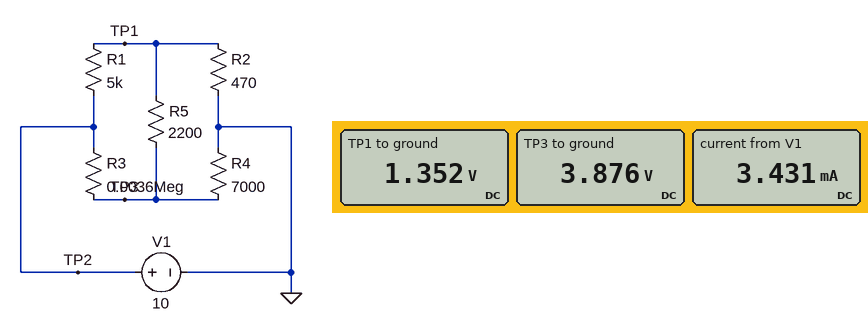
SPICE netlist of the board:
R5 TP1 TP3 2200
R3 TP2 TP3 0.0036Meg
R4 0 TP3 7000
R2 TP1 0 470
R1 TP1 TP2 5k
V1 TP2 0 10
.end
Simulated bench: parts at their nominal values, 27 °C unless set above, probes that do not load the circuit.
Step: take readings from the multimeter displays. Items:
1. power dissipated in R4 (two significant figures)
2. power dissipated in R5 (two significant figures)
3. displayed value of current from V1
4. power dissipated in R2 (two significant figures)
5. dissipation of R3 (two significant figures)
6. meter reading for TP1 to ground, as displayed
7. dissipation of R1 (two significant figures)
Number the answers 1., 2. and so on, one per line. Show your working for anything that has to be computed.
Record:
1. (3.876 V)^2 / 7 kΩ = 2.1 mW
2. (3.876 V - 1.352 V)^2 / 2.2 kΩ = 2.9 mW
3. 3.431 mA
4. (1.352 V)^2 / 470 Ω = 3.9 mW
5. (10 V - 3.876 V)^2 / 3.6 kΩ = 10 mW
6. 1.352 V
7. (10 V - 1.352 V)^2 / 5 kΩ = 15 mW
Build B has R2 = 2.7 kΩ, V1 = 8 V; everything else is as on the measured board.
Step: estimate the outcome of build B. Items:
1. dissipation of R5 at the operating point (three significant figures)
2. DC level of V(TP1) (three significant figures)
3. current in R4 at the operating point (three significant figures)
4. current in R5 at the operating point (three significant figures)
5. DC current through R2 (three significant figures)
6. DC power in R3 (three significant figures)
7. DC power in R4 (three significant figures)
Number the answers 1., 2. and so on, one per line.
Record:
1. 337 µW
2. 3.49 V
3. 622 µA
4. 391 µA
5. 1.29 mA
6. 3.70 mW
7. 2.71 mW
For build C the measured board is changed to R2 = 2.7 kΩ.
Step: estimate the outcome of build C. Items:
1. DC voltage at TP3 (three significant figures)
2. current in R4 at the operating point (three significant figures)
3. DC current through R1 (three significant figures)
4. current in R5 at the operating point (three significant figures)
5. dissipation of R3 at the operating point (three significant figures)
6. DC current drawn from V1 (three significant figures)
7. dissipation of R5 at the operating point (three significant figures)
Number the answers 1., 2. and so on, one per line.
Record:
1. 5.44 V
2. 777 µA
3. 1.13 mA
4. 489 µA
5. 5.77 mW
6. 2.39 mA
7. 527 µW
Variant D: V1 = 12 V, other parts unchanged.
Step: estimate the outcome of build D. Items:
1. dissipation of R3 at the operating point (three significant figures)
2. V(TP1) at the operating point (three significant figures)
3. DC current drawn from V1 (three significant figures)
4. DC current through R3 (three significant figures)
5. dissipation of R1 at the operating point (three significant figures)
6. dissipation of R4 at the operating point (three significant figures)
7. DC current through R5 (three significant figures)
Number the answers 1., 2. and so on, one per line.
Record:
1. 15.0 mW
2. 1.62 V
3. 4.12 mA
4. 2.04 mA
5. 21.5 mW
6. 3.09 mW
7. 1.38 mA
